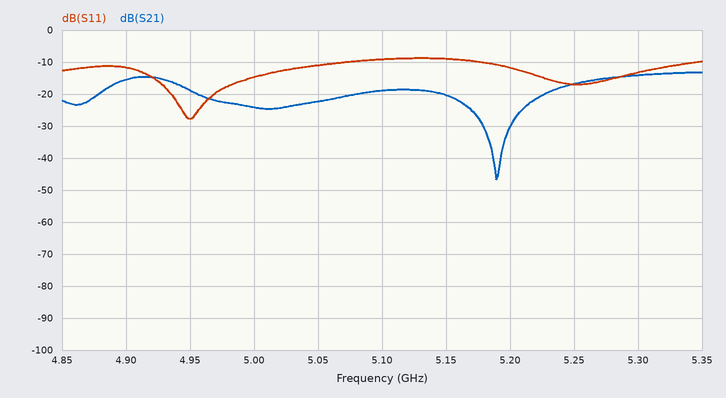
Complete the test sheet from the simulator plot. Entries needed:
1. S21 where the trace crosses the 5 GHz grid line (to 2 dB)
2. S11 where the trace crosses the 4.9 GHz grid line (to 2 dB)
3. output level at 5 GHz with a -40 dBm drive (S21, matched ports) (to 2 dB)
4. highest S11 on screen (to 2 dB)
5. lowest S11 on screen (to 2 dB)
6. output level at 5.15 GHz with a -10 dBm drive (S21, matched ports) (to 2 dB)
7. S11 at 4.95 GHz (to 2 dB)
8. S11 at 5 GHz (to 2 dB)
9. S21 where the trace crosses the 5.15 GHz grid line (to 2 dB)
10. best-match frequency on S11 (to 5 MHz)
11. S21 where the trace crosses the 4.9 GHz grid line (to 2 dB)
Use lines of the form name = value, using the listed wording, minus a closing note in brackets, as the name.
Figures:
S21 where the trace crosses the 5 GHz grid line = -24 dB
S11 where the trace crosses the 4.9 GHz grid line = -12 dB
output level at 5 GHz with a -40 dBm drive (S21, matched ports) = -64 dBm
highest S11 on screen = -8 dB
lowest S11 on screen = -28 dB
output level at 5.15 GHz with a -10 dBm drive (S21, matched ports) = -30 dBm
S11 at 4.95 GHz = -28 dB
S11 at 5 GHz = -14 dB
S21 where the trace crosses the 5.15 GHz grid line = -20 dB
best-match frequency on S11 = 4.950 GHz
S21 where the trace crosses the 4.9 GHz grid line = -16 dB
